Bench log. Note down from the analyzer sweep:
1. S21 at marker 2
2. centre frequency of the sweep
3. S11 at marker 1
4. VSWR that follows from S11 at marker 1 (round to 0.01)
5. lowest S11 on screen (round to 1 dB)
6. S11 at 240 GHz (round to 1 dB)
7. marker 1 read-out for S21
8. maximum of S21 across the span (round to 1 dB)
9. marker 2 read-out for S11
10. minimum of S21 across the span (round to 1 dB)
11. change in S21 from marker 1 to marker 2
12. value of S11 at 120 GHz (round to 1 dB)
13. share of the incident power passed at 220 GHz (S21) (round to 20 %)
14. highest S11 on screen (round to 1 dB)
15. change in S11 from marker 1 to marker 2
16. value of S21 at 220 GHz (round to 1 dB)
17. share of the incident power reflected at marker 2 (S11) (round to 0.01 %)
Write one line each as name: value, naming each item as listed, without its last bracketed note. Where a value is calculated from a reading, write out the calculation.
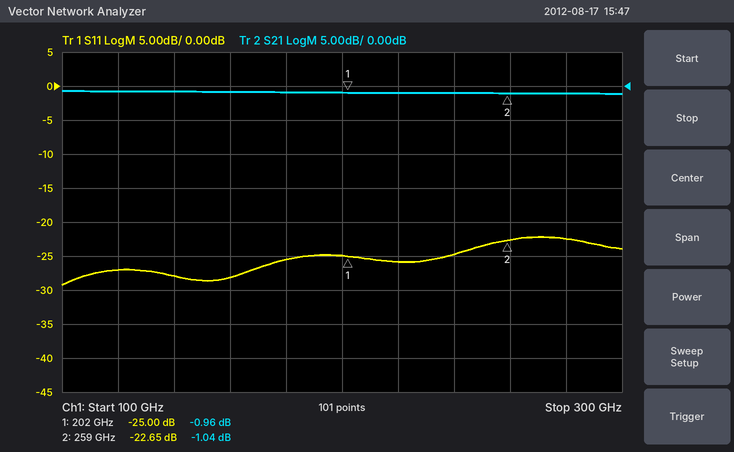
S21 at marker 2: -1.04 dB
centre frequency of the sweep: 200 GHz
S11 at marker 1: -25.00 dB
VSWR that follows from S11 at marker 1: (1 + 0.0562)/(1 − 0.0562) ≈ 1.12
lowest S11 on screen: -29 dB
S11 at 240 GHz: -25 dB
marker 1 read-out for S21: -0.96 dB
maximum of S21 across the span: -1 dB
marker 2 read-out for S11: -22.65 dB
minimum of S21 across the span: -1 dB
change in S21 from marker 1 to marker 2: -1.04 − (-0.96) = -0.08 dB
value of S11 at 120 GHz: -27 dB
share of the incident power passed at 220 GHz (S21): 10^(-1/10) ≈ 79.4 %, so 80 % to the nearest 20 %
highest S11 on screen: -22 dB
change in S11 from marker 1 to marker 2: -22.65 − (-25) = 2.35 dB
value of S21 at 220 GHz: -1 dB
share of the incident power reflected at marker 2 (S11): 10^(-22.65/10) ≈ 0.54 %
